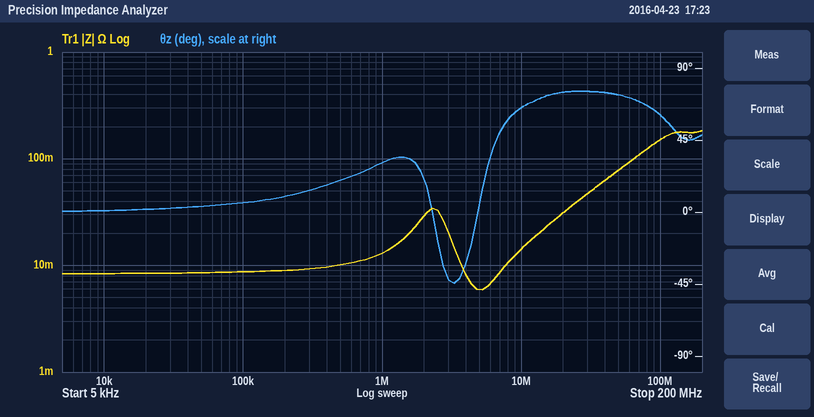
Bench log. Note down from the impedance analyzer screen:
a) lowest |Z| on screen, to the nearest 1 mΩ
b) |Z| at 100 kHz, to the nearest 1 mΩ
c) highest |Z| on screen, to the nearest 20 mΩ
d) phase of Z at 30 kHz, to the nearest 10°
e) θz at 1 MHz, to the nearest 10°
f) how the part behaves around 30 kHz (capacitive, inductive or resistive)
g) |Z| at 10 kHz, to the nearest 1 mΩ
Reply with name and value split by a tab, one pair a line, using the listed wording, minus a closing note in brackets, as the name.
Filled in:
lowest |Z| on screen, to the nearest 1 mΩ	6 mΩ
|Z| at 100 kHz, to the nearest 1 mΩ	9 mΩ
highest |Z| on screen, to the nearest 20 mΩ	180 mΩ
phase of Z at 30 kHz, to the nearest 10°	0°
θz at 1 MHz, to the nearest 10°	30°
how the part behaves around 30 kHz	resistive
|Z| at 10 kHz, to the nearest 1 mΩ	8 mΩ
